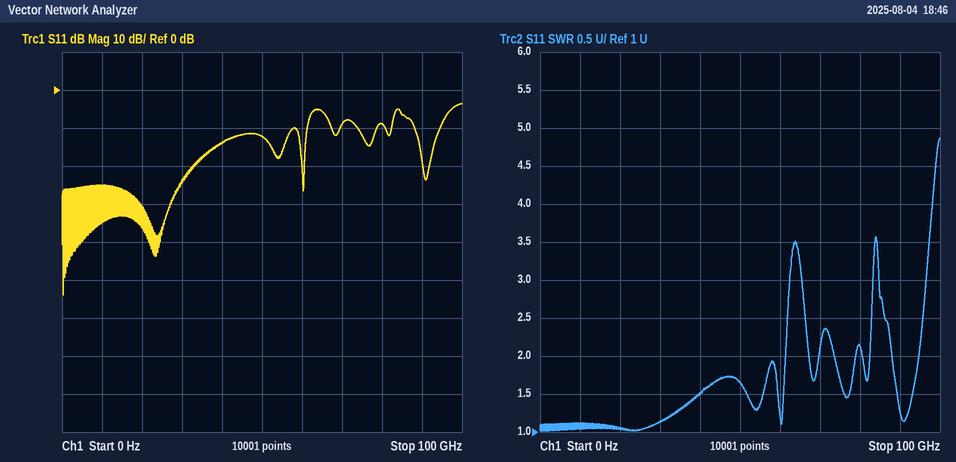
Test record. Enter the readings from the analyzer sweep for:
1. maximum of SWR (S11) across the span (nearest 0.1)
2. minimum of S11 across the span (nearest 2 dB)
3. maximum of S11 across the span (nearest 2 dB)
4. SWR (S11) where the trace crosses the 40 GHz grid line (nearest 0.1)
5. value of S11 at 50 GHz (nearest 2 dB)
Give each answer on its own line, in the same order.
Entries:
4.9
-54 dB
-4 dB
1.5
-12 dB
